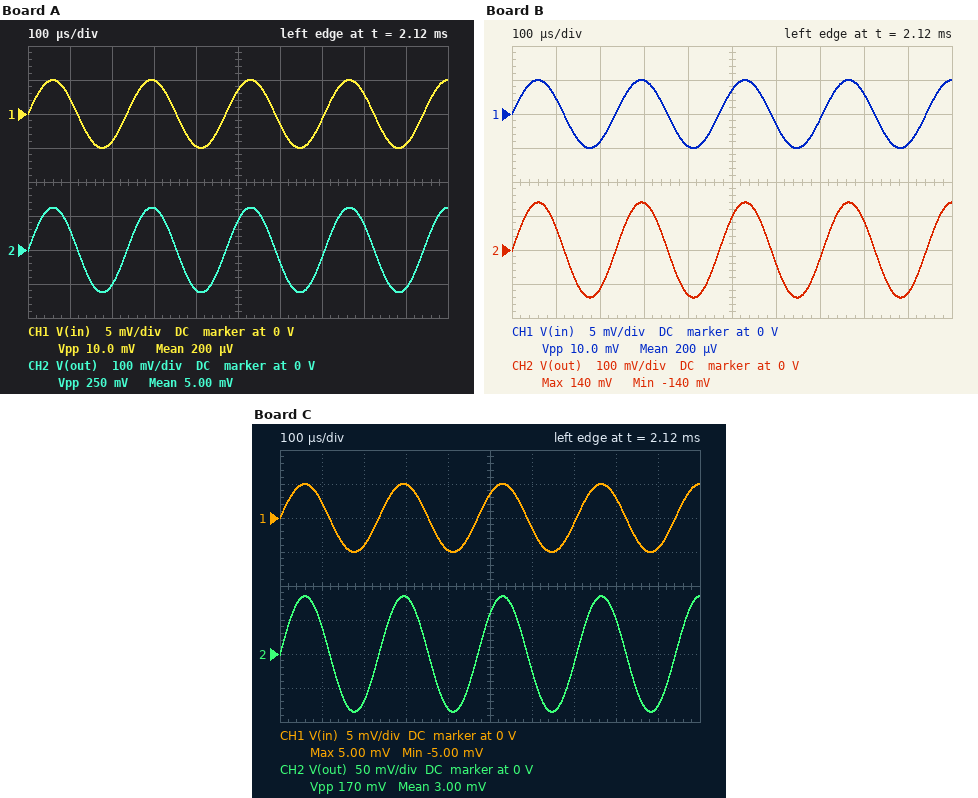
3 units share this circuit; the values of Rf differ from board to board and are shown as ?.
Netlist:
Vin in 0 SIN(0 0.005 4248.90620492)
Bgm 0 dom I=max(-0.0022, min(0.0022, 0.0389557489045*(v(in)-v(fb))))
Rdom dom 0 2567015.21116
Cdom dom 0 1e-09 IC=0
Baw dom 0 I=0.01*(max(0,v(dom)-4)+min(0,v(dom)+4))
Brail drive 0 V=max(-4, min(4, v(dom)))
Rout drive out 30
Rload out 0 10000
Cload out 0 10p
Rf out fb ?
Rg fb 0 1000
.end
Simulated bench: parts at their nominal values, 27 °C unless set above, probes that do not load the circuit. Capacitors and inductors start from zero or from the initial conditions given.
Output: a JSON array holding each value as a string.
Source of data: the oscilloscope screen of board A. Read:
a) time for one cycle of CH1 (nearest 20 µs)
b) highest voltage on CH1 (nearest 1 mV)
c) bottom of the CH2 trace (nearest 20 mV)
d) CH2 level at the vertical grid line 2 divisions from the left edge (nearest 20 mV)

["240 µs", "5 mV", "-120 mV", "-100 mV"]
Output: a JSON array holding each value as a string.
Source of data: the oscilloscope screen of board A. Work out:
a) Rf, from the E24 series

["24 kΩ"]
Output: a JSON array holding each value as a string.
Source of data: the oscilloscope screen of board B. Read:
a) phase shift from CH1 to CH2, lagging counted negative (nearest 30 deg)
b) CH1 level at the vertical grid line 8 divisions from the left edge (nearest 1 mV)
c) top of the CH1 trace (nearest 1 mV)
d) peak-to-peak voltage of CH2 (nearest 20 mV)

["0 deg", "3 mV", "5 mV", "280 mV"]
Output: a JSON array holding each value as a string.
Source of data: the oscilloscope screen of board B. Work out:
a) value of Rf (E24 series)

["27 kΩ"]
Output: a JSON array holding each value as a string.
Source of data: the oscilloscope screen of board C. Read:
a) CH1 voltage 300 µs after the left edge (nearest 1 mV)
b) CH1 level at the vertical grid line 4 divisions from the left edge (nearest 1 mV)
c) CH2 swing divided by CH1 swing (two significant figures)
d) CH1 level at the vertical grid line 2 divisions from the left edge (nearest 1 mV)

["5 mV", "-5 mV", "17", "-4 mV"]
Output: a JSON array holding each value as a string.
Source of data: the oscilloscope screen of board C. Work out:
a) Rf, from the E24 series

["16 kΩ"]
